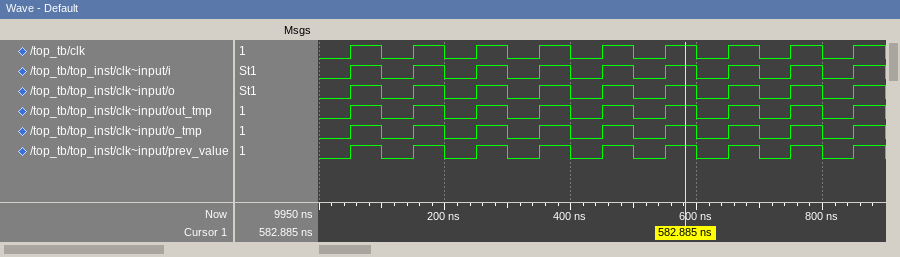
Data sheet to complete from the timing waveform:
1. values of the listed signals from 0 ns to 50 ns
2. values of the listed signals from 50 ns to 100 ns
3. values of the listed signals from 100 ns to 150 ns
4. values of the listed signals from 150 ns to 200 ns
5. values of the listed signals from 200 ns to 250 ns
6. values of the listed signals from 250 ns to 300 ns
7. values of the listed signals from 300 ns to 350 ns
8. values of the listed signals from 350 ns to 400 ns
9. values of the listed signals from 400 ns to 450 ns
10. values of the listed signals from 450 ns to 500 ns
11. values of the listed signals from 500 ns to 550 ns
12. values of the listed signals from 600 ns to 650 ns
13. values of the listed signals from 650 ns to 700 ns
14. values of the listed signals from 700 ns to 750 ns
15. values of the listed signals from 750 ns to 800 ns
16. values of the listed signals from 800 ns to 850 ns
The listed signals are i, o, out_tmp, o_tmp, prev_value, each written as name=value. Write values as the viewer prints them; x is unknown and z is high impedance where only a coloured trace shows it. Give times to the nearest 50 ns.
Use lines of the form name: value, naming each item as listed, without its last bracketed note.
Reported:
values of the listed signals from 0 ns to 50 ns: i=0, o=0, out_tmp=0, o_tmp=0, prev_value=0
values of the listed signals from 50 ns to 100 ns: i=1, o=1, out_tmp=1, o_tmp=1, prev_value=1
values of the listed signals from 100 ns to 150 ns: i=0, o=0, out_tmp=0, o_tmp=0, prev_value=0
values of the listed signals from 150 ns to 200 ns: i=1, o=1, out_tmp=1, o_tmp=1, prev_value=1
values of the listed signals from 200 ns to 250 ns: i=0, o=0, out_tmp=0, o_tmp=0, prev_value=0
values of the listed signals from 250 ns to 300 ns: i=1, o=1, out_tmp=1, o_tmp=1, prev_value=1
values of the listed signals from 300 ns to 350 ns: i=0, o=0, out_tmp=0, o_tmp=0, prev_value=0
values of the listed signals from 350 ns to 400 ns: i=1, o=1, out_tmp=1, o_tmp=1, prev_value=1
values of the listed signals from 400 ns to 450 ns: i=0, o=0, out_tmp=0, o_tmp=0, prev_value=0
values of the listed signals from 450 ns to 500 ns: i=1, o=1, out_tmp=1, o_tmp=1, prev_value=1
values of the listed signals from 500 ns to 550 ns: i=0, o=0, out_tmp=0, o_tmp=0, prev_value=0
values of the listed signals from 600 ns to 650 ns: i=0, o=0, out_tmp=0, o_tmp=0, prev_value=0
values of the listed signals from 650 ns to 700 ns: i=1, o=1, out_tmp=1, o_tmp=1, prev_value=1
values of the listed signals from 700 ns to 750 ns: i=0, o=0, out_tmp=0, o_tmp=0, prev_value=0
values of the listed signals from 750 ns to 800 ns: i=1, o=1, out_tmp=1, o_tmp=1, prev_value=1
values of the listed signals from 800 ns to 850 ns: i=0, o=0, out_tmp=0, o_tmp=0, prev_value=0
